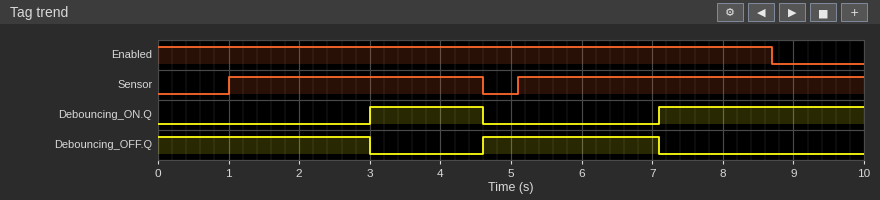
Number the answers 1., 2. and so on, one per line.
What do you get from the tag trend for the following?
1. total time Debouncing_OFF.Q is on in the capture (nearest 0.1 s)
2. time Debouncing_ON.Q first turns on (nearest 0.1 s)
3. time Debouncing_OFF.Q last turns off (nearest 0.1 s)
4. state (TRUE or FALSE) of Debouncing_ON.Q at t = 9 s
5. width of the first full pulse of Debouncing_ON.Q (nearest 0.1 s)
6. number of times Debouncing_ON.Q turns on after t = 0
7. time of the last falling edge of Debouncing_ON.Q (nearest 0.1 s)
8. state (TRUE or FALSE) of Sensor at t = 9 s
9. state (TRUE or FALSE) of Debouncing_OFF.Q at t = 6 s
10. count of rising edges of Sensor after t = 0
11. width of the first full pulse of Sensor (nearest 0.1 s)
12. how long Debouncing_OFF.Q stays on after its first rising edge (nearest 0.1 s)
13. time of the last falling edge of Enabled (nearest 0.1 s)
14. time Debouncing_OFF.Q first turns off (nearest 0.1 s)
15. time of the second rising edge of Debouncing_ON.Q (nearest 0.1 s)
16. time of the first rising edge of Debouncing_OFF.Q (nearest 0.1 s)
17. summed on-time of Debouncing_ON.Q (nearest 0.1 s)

1. 5.5 s
2. 3.0 s
3. 7.1 s
4. TRUE
5. 1.6 s
6. 2
7. 4.6 s
8. TRUE
9. TRUE
10. 2
11. 3.6 s
12. 2.5 s
13. 8.7 s
14. 3.0 s
15. 7.1 s
16. 4.6 s
17. 4.5 s
